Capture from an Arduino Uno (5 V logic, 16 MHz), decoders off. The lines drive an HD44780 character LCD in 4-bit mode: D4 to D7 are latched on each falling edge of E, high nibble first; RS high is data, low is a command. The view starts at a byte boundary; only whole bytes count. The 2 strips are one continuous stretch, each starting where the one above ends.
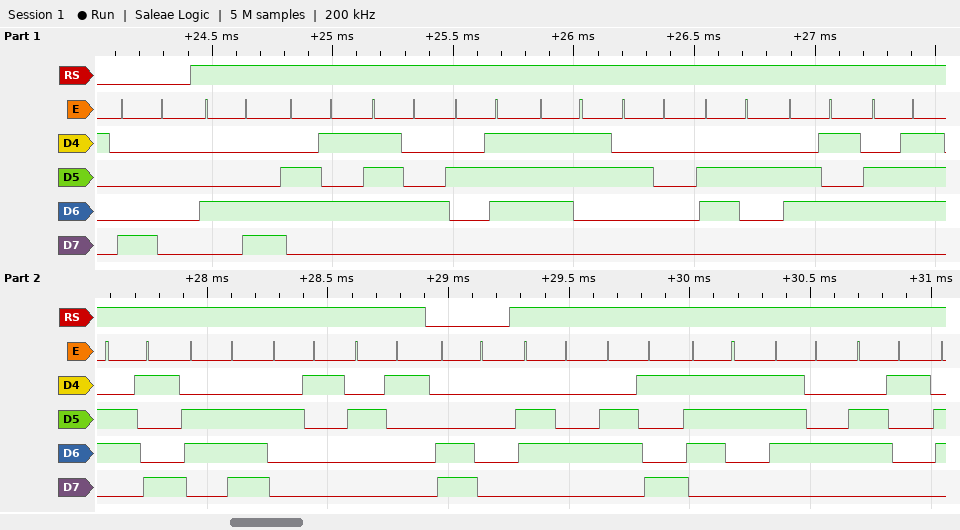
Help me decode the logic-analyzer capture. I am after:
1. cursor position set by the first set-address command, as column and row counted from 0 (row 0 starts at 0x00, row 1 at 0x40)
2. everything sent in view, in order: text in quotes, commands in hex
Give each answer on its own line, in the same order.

column 0, row 0
0x80 "Let's begin!!" 0xC0 "dista"
